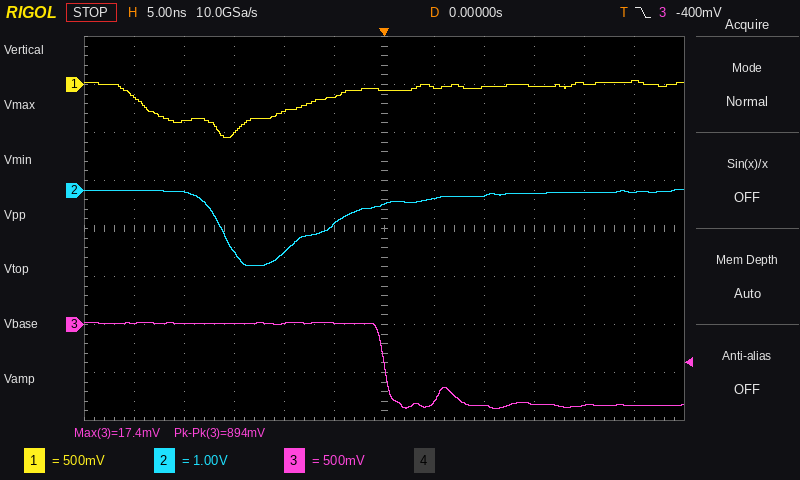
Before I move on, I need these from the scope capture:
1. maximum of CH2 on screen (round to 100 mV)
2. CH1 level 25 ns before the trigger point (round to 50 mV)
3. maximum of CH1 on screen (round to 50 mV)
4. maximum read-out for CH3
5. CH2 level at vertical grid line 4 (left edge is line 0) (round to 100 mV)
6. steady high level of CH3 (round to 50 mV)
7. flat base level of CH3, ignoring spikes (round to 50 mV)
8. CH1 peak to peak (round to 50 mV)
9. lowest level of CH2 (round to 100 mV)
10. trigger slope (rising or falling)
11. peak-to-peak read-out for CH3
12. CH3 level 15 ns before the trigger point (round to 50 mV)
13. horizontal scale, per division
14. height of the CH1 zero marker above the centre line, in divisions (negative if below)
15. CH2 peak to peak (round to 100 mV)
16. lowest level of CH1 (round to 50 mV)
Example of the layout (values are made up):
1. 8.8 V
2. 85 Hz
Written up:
1. 0.0 V
2. -150 mV
3. 50 mV
4. 17.4 mV
5. -1.3 V
6. 0 mV
7. -850 mV
8. 600 mV
9. -1.6 V
10. falling
11. 894 mV
12. 0 mV
13. 5 ns
14. +3.0 div
15. 1.6 V
16. -550 mV
